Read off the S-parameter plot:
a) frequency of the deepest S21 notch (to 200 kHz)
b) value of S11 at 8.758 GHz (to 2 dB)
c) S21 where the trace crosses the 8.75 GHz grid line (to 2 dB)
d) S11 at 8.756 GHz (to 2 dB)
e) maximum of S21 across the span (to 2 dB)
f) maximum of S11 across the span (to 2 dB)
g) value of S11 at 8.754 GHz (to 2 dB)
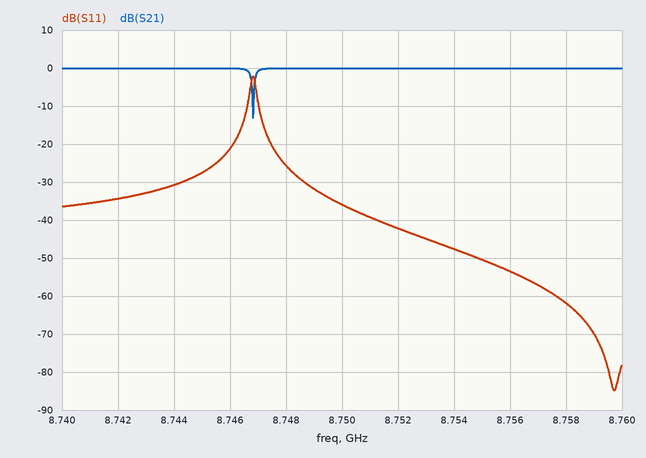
8.7468 GHz
-62 dB
0 dB
-54 dB
0 dB
-2 dB
-48 dB
